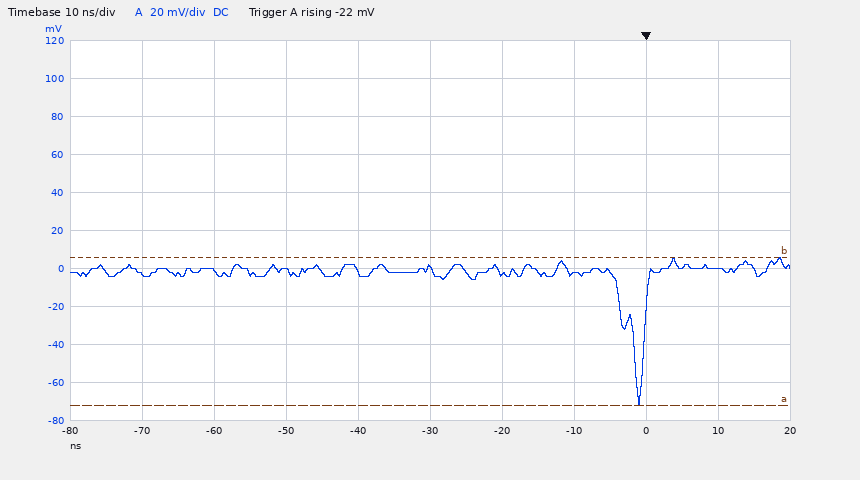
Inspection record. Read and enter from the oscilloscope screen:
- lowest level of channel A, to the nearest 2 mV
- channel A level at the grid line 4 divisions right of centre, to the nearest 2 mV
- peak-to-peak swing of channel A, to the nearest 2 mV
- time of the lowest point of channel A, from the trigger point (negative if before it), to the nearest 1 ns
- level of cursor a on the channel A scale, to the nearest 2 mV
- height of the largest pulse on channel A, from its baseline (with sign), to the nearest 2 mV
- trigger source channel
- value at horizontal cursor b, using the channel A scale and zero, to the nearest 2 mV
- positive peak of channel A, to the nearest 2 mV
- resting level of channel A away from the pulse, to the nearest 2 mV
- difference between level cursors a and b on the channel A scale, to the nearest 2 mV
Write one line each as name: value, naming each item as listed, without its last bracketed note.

lowest level of channel A, to the nearest 2 mV: -72 mV
channel A level at the grid line 4 divisions right of centre, to the nearest 2 mV: 0 mV
peak-to-peak swing of channel A, to the nearest 2 mV: 78 mV
time of the lowest point of channel A, from the trigger point (negative if before it), to the nearest 1 ns: -1 ns
level of cursor a on the channel A scale, to the nearest 2 mV: -72 mV
height of the largest pulse on channel A, from its baseline (with sign), to the nearest 2 mV: -70 mV
trigger source channel: channel A
value at horizontal cursor b, using the channel A scale and zero, to the nearest 2 mV: 6 mV
positive peak of channel A, to the nearest 2 mV: 6 mV
resting level of channel A away from the pulse, to the nearest 2 mV: -2 mV
difference between level cursors a and b on the channel A scale, to the nearest 2 mV: 78 mV
